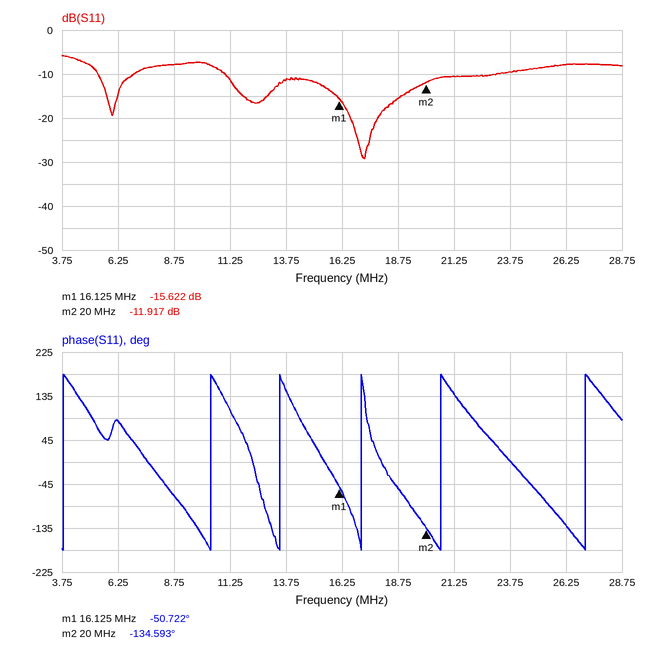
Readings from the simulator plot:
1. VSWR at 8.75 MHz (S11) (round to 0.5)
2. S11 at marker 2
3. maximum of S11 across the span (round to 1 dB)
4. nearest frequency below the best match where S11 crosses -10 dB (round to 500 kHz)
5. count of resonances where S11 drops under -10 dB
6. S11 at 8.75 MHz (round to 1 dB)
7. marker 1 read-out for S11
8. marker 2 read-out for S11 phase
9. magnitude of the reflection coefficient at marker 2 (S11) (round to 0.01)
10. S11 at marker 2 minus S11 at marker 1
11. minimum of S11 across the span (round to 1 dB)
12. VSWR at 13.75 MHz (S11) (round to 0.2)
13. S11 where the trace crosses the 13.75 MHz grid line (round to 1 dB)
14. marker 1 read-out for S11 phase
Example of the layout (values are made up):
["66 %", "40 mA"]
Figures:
["2.5", "-11.917 dB", "-6 dB", "11.0 MHz", "3", "-8 dB", "-15.622 dB", "-134.593°", "0.25", "3.705 dB", "-29 dB", "1.8", "-11 dB", "-50.722°"]
